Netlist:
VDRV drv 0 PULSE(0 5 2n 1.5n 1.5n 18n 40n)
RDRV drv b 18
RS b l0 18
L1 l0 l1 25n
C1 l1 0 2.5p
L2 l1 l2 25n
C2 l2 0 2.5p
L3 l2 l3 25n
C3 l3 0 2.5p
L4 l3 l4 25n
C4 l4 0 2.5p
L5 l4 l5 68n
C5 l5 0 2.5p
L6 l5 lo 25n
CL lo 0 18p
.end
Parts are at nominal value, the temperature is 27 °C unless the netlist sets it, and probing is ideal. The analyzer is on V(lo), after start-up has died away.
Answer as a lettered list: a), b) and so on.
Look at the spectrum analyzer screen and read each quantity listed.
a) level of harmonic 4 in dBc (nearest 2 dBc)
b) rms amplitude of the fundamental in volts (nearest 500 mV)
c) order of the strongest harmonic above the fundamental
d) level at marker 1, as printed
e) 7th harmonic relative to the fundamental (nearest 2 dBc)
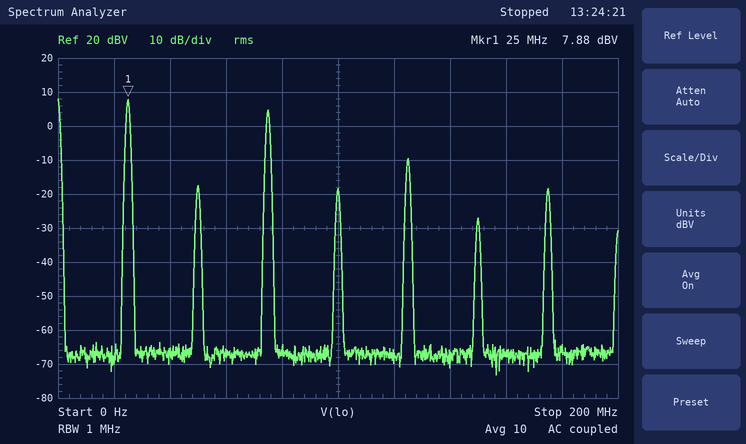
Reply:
a) -26 dBc
b) 2.5 V
c) 3
d) 7.88 dBV
e) -26 dBc
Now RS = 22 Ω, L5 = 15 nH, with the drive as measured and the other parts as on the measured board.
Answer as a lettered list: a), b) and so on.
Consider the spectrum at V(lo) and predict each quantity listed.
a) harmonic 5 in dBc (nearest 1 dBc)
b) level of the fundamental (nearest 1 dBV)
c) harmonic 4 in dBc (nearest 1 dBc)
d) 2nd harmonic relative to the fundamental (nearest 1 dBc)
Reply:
a) -15 dBc
b) 8 dBV
c) -25 dBc
d) -26 dBc
